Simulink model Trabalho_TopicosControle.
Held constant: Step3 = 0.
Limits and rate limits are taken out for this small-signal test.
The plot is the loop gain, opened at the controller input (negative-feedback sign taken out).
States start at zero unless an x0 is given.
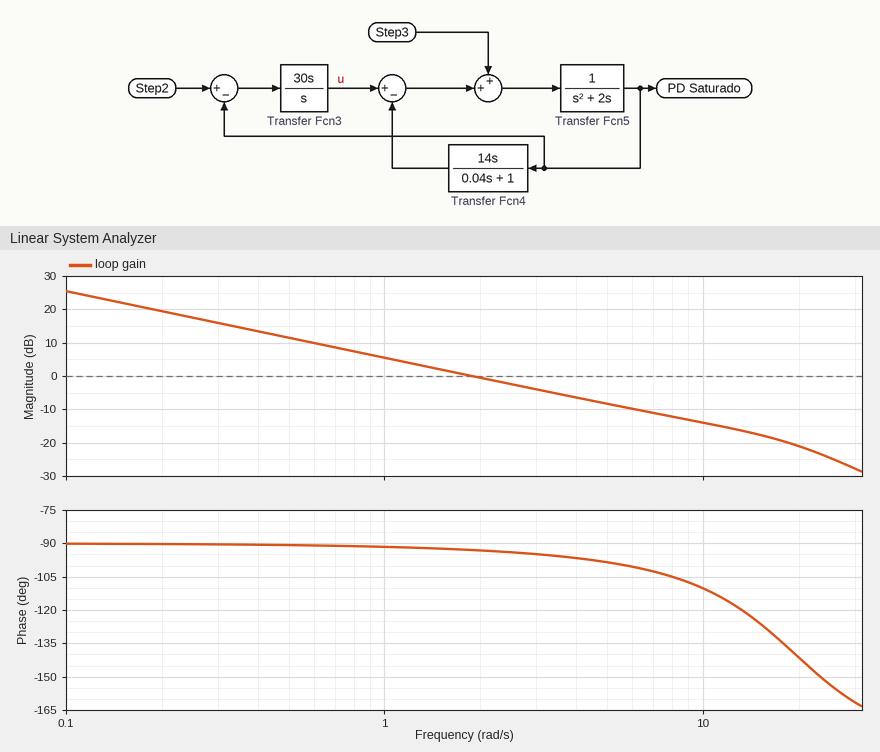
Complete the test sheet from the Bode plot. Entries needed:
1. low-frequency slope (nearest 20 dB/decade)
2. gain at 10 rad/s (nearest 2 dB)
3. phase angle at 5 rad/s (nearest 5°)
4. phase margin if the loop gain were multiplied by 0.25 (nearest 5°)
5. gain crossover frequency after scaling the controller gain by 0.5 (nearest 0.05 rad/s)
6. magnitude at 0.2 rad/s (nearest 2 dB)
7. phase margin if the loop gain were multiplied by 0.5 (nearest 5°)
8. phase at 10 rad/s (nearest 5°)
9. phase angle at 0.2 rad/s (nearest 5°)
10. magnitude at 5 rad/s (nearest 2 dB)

-20 dB/decade
-14 dB
-100°
90°
0.95 rad/s
20 dB
90°
-110°
-90°
-8 dB
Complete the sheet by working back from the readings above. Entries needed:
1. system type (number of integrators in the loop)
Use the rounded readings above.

1
